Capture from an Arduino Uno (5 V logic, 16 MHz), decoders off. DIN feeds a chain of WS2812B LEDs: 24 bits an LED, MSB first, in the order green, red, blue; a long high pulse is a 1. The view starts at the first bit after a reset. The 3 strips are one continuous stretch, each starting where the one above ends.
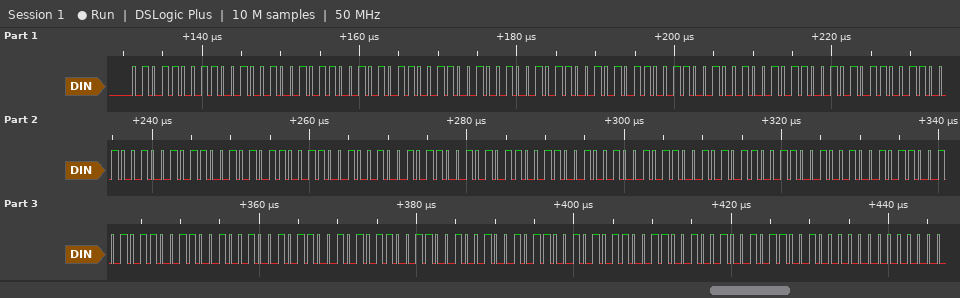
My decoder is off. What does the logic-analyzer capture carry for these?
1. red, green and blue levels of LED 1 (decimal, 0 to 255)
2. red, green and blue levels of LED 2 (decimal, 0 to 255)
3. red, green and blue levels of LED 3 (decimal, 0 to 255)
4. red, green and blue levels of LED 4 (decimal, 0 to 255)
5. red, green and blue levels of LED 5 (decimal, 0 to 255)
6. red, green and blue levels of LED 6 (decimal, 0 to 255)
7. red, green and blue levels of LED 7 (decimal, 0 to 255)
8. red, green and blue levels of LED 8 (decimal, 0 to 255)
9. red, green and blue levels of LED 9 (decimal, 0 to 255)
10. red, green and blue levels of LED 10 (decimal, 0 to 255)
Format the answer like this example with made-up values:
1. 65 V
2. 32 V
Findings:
1. 146, 89, 89
2. 146, 89, 89
3. 146, 89, 89
4. 146, 89, 89
5. 146, 89, 89
6. 146, 89, 89
7. 146, 89, 89
8. 146, 89, 89
9. 146, 89, 89
10. 146, 89, 89
